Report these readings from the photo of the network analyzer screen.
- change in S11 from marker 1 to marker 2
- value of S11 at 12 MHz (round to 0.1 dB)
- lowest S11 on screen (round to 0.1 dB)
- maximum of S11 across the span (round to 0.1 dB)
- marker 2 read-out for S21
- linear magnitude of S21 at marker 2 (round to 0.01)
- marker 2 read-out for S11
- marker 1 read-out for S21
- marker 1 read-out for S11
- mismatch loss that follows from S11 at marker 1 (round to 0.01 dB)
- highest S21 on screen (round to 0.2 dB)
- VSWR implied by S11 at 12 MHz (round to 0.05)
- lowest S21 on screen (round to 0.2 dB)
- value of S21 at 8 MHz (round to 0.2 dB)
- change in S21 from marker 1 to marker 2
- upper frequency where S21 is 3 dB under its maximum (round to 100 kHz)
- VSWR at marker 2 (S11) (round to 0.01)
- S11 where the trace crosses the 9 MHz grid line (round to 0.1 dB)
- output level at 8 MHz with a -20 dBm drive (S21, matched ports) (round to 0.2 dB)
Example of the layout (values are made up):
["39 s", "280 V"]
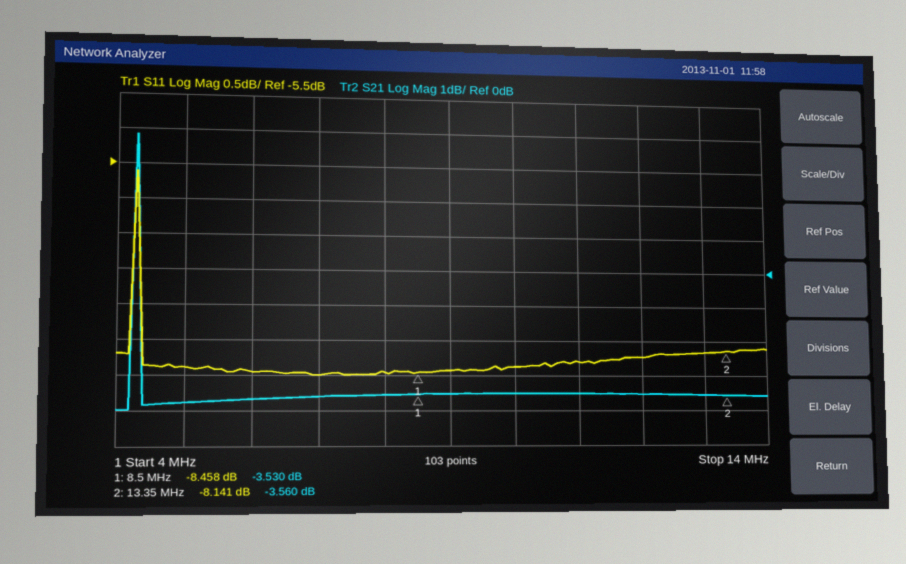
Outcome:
["0.317 dB", "-8.2 dB", "-8.5 dB", "-5.6 dB", "-3.560 dB", "0.66", "-8.141 dB", "-3.530 dB", "-8.458 dB", "0.67 dB", "3.8 dB", "2.25", "-4.0 dB", "-3.6 dB", "-0.030 dB", "4.3 MHz", "2.29", "-8.4 dB", "-23.6 dBm"]
